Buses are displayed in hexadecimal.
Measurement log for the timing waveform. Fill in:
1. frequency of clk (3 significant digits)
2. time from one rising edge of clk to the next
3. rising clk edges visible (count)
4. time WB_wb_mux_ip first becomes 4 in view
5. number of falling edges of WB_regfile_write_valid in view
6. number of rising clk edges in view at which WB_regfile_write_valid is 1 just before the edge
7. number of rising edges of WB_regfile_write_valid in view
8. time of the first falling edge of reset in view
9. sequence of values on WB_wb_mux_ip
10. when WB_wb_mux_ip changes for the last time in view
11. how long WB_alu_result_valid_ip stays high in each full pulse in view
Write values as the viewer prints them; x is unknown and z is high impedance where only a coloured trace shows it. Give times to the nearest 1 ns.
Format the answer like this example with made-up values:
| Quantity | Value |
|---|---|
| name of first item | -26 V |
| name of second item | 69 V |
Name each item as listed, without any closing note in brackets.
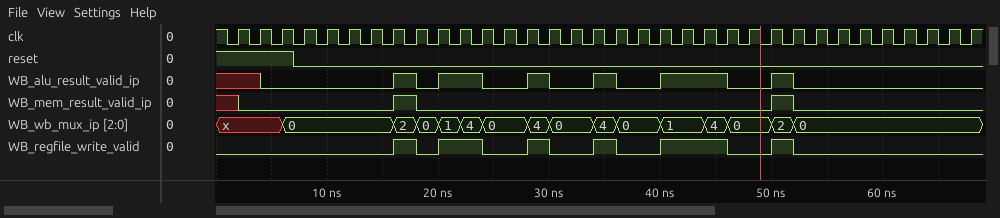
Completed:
| Quantity | Value |
|---|---|
| frequency of clk | 500 MHz |
| time from one rising edge of clk to the next | 2 ns |
| rising clk edges visible | 34 |
| time WB_wb_mux_ip first becomes 4 in view | 22 ns |
| number of falling edges of WB_regfile_write_valid in view | 6 |
| number of rising clk edges in view at which WB_regfile_write_valid is 1 just before the edge | 9 |
| number of rising edges of WB_regfile_write_valid in view | 6 |
| time of the first falling edge of reset in view | 7 ns |
| sequence of values on WB_wb_mux_ip | x, 0, 2, 0, 1, 4, 0, 4, 0, 4, 0, 1, 4, 0, 2, 0 |
| when WB_wb_mux_ip changes for the last time in view | 52 ns |
| how long WB_alu_result_valid_ip stays high in each full pulse in view | 2 ns, 4 ns, 2 ns, 2 ns, 6 ns, 2 ns |
